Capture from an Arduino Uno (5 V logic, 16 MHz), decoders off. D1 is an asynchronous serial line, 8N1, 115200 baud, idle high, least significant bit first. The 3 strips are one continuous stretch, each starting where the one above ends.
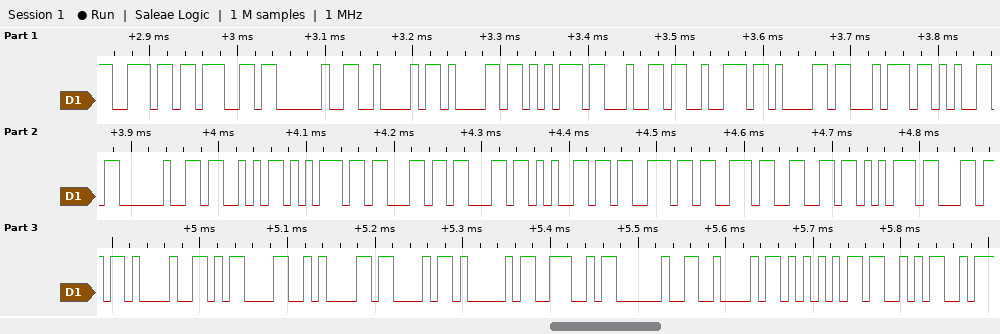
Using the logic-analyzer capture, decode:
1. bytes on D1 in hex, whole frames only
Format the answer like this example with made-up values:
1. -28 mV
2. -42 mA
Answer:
1. 6E 67 20 42 61 75 64 72 61 74 65 20 53 75 63 63 65 73 73 66 75 6C 21 0D 0A 43 41 4E 20 42 55 53
